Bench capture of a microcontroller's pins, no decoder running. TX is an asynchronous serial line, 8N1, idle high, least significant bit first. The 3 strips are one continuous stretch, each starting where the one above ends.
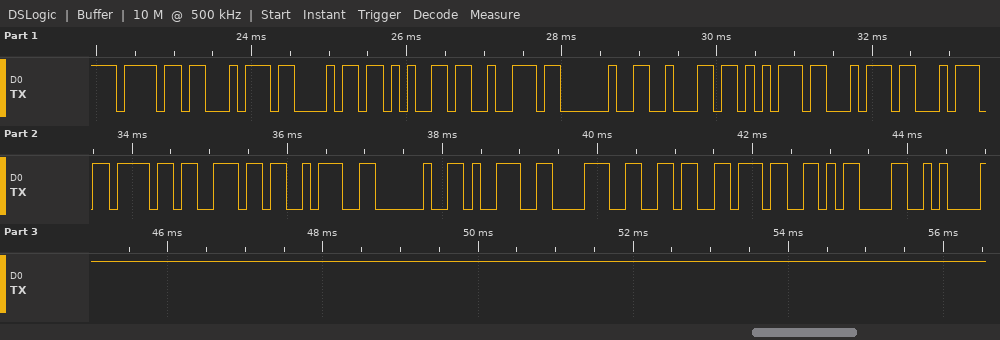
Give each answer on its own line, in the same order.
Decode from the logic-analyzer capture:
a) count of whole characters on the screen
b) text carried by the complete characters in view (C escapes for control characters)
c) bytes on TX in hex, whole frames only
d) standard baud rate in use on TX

20
"other button: 9867\r\n"
6F 74 68 65 72 20 62 75 74 74 6F 6E 3A 20 39 38 36 37 0D 0A
9600 baud
